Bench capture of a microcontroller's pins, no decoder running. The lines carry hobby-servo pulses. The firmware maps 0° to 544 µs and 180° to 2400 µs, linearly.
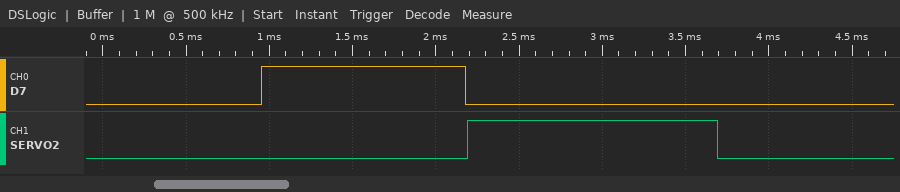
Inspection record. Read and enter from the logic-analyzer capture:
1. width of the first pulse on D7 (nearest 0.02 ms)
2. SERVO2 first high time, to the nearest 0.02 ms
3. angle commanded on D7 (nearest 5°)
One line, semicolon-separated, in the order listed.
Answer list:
1.22 ms; 1.50 ms; 65°
